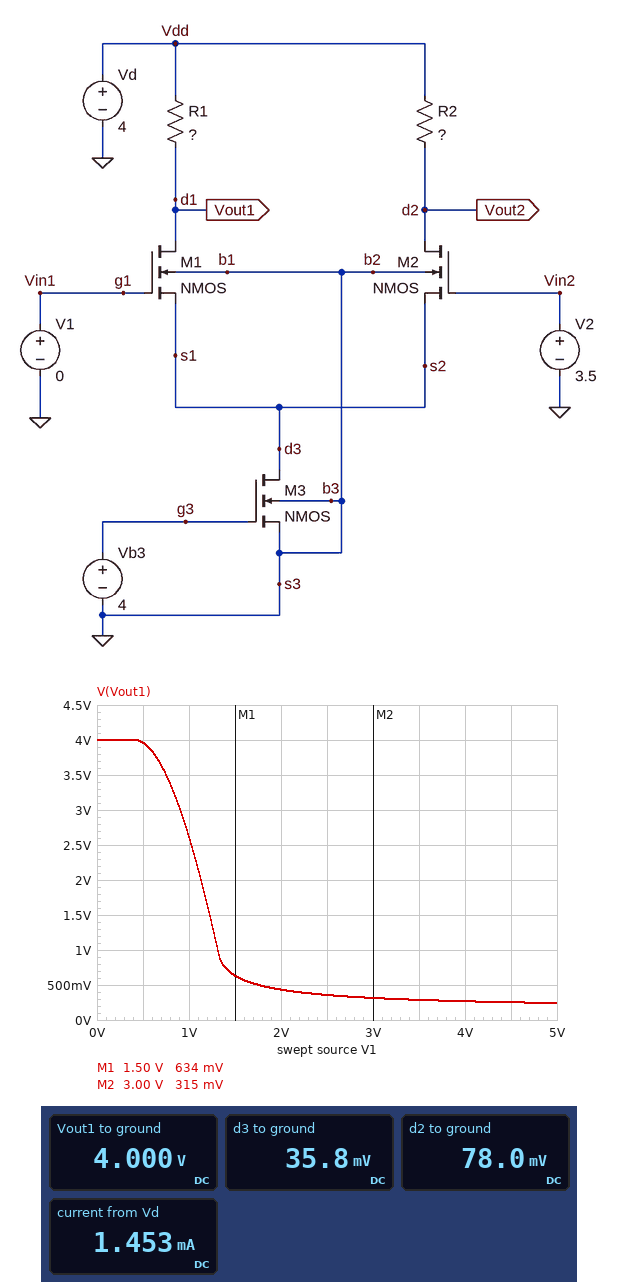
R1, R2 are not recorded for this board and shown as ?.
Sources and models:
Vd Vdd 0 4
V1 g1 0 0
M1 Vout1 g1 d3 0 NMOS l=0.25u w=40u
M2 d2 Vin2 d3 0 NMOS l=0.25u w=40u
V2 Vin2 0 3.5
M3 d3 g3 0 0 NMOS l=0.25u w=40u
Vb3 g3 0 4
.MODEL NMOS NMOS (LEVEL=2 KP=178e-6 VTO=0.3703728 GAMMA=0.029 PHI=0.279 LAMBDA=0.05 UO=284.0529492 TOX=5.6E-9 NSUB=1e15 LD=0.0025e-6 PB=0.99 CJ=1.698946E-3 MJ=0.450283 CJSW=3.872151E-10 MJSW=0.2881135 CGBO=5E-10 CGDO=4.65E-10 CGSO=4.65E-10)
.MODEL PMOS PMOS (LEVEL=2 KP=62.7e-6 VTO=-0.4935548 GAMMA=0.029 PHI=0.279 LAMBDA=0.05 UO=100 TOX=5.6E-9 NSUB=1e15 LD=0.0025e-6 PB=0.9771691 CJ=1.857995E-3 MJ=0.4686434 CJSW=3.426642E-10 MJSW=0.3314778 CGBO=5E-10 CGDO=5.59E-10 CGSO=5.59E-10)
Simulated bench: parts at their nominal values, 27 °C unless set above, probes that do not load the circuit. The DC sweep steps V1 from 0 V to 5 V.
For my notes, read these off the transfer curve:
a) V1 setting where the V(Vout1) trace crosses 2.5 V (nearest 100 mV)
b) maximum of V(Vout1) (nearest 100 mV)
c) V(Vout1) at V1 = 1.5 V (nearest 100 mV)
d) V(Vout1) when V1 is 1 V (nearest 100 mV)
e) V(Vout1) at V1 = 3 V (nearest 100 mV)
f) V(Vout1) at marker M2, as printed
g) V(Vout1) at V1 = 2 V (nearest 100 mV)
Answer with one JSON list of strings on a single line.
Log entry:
["1.0 V", "4.0 V", "600 mV", "2.6 V", "300 mV", "315 mV", "400 mV"]
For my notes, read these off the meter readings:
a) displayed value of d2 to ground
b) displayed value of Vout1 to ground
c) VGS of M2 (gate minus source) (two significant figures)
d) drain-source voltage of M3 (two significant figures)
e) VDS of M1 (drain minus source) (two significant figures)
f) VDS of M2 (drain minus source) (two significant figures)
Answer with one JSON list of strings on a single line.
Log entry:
["78.0 mV", "4.000 V", "3.5 V", "36 mV", "4.0 V", "42 mV"]
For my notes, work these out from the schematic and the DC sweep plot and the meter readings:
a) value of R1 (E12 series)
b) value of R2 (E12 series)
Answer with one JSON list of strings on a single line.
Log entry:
["820 Ω", "2.7 kΩ"]
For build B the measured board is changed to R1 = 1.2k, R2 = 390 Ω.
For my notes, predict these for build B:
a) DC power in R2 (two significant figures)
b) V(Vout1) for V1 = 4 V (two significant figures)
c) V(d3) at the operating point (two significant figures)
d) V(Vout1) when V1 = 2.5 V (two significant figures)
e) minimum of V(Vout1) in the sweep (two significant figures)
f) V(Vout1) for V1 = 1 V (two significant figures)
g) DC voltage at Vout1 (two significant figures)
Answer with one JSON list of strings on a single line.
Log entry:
["31 mW", "380 mV", "230 mV", "450 mV", "360 mV", "3.0 V", "4.0 V"]
